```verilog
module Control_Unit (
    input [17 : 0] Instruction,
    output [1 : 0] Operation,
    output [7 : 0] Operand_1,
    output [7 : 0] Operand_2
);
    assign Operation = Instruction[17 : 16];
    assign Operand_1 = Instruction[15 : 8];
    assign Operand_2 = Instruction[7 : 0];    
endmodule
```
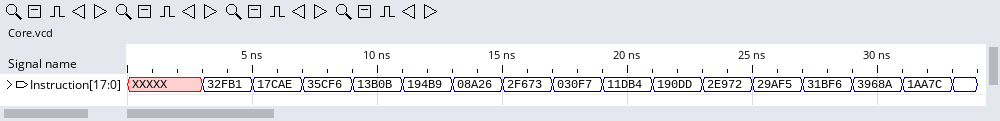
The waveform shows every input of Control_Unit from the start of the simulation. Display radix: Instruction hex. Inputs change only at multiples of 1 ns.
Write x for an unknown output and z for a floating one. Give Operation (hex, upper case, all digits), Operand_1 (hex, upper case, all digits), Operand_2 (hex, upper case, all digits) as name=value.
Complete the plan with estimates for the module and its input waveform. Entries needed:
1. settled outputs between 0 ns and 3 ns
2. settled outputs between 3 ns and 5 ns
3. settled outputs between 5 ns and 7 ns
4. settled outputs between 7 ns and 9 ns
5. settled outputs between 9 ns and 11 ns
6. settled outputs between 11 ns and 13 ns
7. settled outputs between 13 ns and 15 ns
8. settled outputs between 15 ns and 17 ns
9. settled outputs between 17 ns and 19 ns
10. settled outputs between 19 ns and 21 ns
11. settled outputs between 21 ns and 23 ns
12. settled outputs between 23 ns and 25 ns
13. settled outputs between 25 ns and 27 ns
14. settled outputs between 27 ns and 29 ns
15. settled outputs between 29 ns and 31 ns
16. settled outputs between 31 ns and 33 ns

Operation=x, Operand_1=x, Operand_2=x
Operation=3, Operand_1=2F, Operand_2=B1
Operation=1, Operand_1=7C, Operand_2=AE
Operation=3, Operand_1=5C, Operand_2=F6
Operation=1, Operand_1=3B, Operand_2=0B
Operation=1, Operand_1=94, Operand_2=B9
Operation=0, Operand_1=8A, Operand_2=26
Operation=2, Operand_1=F6, Operand_2=73
Operation=0, Operand_1=30, Operand_2=F7
Operation=1, Operand_1=1D, Operand_2=B4
Operation=1, Operand_1=90, Operand_2=DD
Operation=2, Operand_1=E9, Operand_2=72
Operation=2, Operand_1=9A, Operand_2=F5
Operation=3, Operand_1=1B, Operand_2=F6
Operation=3, Operand_1=96, Operand_2=8A
Operation=1, Operand_1=AA, Operand_2=7C
